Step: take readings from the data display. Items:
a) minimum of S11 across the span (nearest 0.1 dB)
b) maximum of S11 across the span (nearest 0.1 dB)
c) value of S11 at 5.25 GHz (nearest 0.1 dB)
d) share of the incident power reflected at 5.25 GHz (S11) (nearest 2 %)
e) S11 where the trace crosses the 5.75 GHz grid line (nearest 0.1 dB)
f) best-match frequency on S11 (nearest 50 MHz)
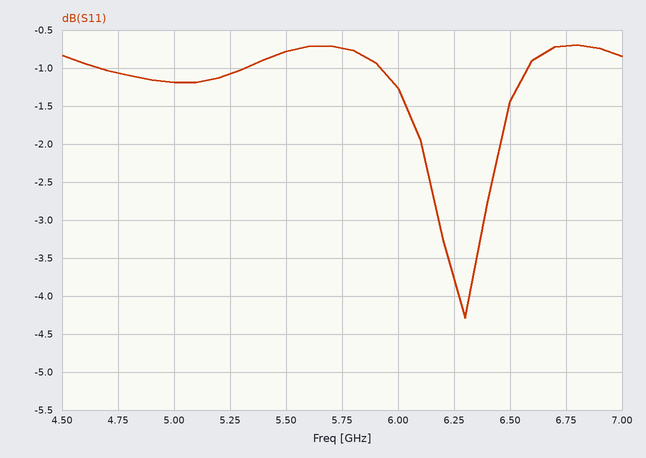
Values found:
-4.3 dB
-0.7 dB
-1.1 dB
78 %
-0.7 dB
6.30 GHz
